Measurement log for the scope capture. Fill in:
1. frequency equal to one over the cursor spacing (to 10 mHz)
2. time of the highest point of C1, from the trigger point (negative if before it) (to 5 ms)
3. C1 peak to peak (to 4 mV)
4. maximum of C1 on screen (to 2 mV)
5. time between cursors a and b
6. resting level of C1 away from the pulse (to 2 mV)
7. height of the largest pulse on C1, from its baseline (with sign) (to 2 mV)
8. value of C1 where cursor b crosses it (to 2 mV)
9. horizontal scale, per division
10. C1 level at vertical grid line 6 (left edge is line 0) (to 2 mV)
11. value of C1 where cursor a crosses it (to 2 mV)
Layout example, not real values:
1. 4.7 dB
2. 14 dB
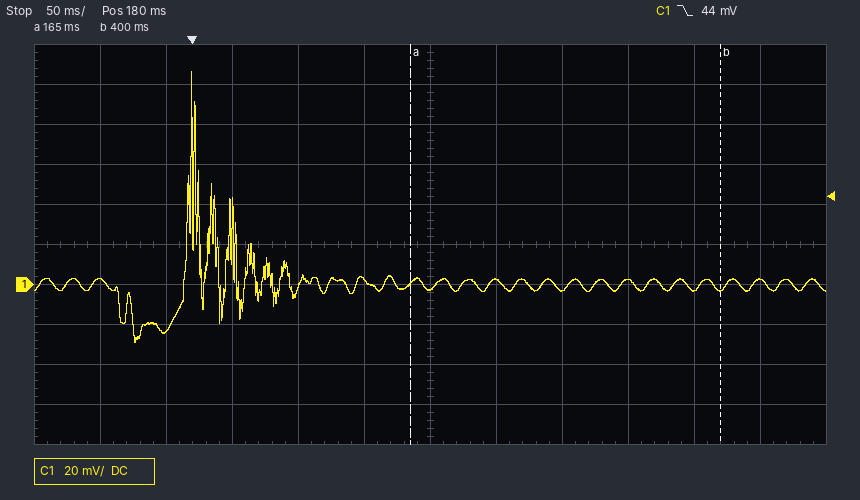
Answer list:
1. 4.26 Hz
2. 0 ms
3. 136 mV
4. 106 mV
5. 235 ms
6. 0 mV
7. +106 mV
8. -2 mV
9. 50 ms
10. -2 mV
11. 0 mV
